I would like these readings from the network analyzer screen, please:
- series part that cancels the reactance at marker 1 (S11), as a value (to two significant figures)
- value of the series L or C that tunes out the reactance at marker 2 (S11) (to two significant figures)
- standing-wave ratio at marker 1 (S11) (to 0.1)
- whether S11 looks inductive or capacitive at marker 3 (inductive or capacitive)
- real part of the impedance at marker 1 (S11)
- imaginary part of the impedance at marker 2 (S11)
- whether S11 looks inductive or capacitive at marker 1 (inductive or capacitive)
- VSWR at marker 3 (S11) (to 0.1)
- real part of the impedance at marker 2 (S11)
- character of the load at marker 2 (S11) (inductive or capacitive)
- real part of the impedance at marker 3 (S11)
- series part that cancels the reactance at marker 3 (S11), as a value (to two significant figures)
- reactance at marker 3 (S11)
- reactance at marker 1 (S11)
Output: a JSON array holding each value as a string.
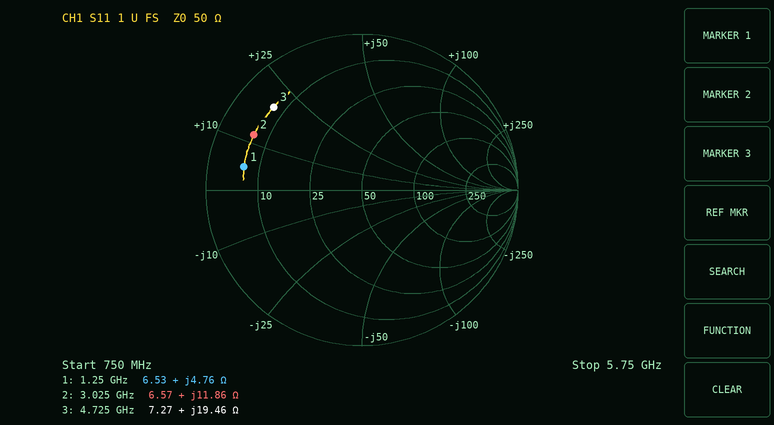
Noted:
["27 pF", "4.4 pF", "7.7", "inductive", "6.53 Ω", "+11.86 Ω", "inductive", "7.9", "6.57 Ω", "inductive", "7.27 Ω", "1.7 pF", "+19.46 Ω", "+4.76 Ω"]
